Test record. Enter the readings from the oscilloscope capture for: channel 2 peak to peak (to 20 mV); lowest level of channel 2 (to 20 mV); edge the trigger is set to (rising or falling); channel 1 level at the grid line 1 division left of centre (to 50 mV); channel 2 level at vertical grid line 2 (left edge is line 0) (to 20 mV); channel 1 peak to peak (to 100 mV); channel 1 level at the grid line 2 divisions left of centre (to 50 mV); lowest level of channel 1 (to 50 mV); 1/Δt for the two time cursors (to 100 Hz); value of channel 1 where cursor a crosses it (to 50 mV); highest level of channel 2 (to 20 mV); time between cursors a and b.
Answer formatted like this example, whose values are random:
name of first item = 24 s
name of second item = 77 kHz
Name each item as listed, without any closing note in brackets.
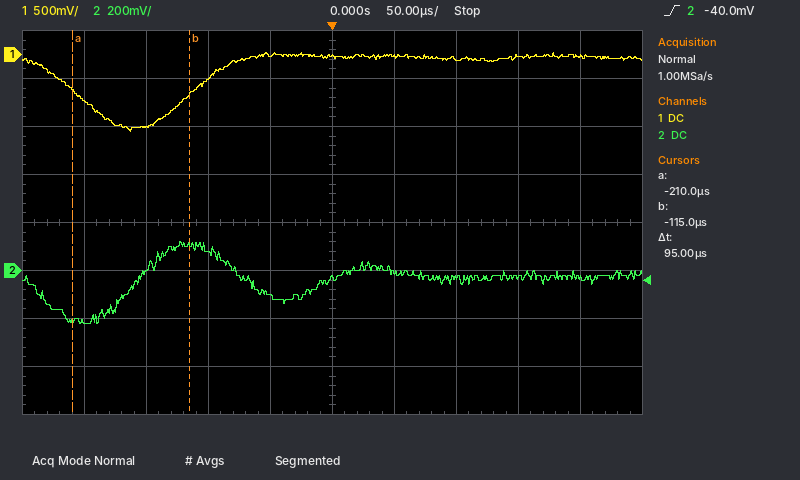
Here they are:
channel 2 peak to peak = 340 mV
lowest level of channel 2 = -220 mV
edge the trigger is set to = rising
channel 1 level at the grid line 1 division left of centre = 0 mV
channel 2 level at vertical grid line 2 (left edge is line 0) = 0 mV
channel 1 peak to peak = 800 mV
channel 1 level at the grid line 2 divisions left of centre = -250 mV
lowest level of channel 1 = -800 mV
1/Δt for the two time cursors = 10.5 kHz
value of channel 1 where cursor a crosses it = -350 mV
highest level of channel 2 = 120 mV
time between cursors a and b = 95 µs
